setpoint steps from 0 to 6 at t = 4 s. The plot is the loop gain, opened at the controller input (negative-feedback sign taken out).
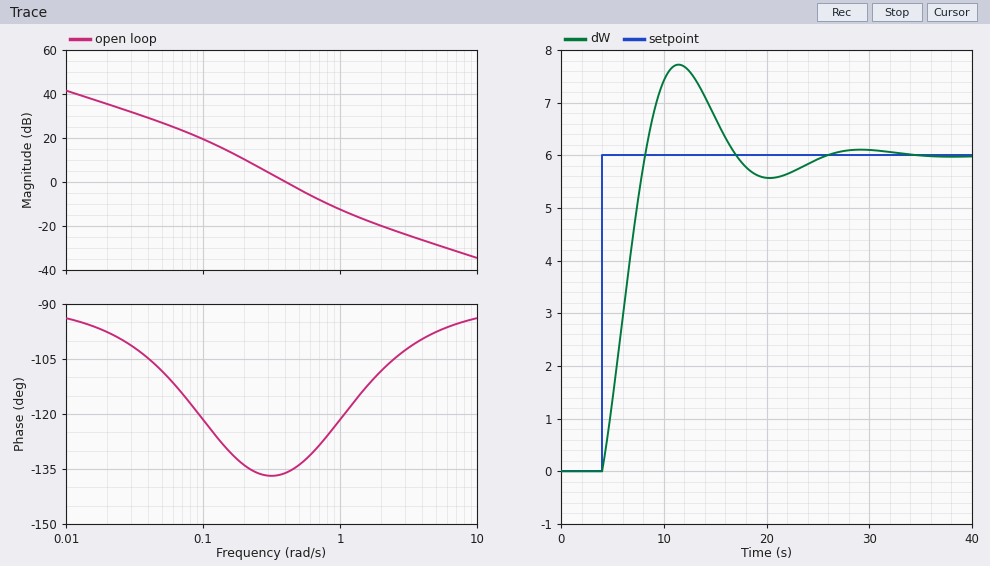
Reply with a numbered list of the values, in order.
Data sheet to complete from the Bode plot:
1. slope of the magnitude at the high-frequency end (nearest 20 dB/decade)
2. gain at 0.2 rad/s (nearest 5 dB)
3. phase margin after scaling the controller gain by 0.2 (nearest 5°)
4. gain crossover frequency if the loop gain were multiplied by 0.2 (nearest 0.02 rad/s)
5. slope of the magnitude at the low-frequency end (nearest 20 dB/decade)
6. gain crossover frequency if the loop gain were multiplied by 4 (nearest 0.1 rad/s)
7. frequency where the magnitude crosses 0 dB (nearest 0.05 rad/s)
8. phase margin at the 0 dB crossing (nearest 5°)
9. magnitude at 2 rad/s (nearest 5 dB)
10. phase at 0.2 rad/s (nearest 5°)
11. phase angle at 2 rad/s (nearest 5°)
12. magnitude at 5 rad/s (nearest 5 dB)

1. -20 dB/decade
2. 10 dB
3. 50°
4. 0.16 rad/s
5. -20 dB/decade
6. 1.0 rad/s
7. 0.40 rad/s
8. 45°
9. -20 dB
10. -135°
11. -110°
12. -30 dB
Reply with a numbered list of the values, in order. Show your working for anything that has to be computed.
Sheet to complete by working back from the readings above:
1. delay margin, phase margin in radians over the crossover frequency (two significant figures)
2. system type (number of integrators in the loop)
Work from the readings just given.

1. 45 × π / 180 / 0.4 = 2.0 s
2. 1
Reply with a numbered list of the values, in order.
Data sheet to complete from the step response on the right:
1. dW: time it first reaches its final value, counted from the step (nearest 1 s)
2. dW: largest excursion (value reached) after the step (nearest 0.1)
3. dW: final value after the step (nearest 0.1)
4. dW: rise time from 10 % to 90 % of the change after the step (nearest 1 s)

1. 4 s
2. 7.7
3. 6.0
4. 3 s
